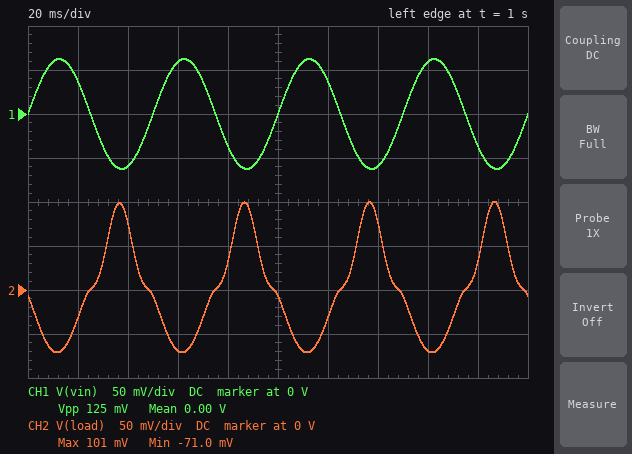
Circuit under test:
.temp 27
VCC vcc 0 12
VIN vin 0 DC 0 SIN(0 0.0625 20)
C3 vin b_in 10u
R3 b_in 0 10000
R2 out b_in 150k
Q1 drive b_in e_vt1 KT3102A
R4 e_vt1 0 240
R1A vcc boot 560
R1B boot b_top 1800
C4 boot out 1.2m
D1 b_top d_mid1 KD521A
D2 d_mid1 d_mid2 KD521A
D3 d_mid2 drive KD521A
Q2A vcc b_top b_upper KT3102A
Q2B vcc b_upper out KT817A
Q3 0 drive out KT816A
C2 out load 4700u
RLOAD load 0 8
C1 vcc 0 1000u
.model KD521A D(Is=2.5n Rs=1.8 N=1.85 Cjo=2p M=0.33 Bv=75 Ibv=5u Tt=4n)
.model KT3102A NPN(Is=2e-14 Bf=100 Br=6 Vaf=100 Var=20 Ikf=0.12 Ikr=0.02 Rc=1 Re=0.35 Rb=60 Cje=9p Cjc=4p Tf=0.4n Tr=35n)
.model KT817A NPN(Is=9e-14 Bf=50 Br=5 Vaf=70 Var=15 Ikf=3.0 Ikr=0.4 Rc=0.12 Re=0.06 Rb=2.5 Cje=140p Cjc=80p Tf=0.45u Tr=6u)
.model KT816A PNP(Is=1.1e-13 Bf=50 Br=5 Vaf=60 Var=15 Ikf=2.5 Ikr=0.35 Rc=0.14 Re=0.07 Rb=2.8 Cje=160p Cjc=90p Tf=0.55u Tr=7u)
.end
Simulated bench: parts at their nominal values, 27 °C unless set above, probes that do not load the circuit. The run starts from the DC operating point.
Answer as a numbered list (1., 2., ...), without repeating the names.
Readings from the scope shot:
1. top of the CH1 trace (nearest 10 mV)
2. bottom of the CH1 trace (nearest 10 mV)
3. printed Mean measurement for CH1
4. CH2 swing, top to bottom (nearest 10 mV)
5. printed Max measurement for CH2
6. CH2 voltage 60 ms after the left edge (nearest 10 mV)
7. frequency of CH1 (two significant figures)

1. 60 mV
2. -60 mV
3. 0.00 V
4. 170 mV
5. 101 mV
6. -70 mV
7. 20 Hz
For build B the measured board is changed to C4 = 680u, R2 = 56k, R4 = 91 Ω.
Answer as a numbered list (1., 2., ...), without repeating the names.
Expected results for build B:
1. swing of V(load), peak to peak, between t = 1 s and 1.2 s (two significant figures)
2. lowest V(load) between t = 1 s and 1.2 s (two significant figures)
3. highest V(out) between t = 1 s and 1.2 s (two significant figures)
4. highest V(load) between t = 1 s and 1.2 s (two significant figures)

1. 1.3 V
2. -380 mV
3. 7.8 V
4. 970 mV
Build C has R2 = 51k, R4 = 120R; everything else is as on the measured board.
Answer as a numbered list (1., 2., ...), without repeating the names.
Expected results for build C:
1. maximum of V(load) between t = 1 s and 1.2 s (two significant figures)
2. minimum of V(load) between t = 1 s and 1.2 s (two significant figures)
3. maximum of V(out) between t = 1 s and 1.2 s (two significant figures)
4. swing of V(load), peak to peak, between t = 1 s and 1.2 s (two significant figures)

1. 560 mV
2. -280 mV
3. 7.2 V
4. 840 mV
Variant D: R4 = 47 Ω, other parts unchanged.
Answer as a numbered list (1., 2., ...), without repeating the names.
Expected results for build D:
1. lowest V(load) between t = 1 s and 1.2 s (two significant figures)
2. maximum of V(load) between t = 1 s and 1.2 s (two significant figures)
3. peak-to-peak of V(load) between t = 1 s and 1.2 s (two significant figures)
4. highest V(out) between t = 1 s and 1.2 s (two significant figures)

1. -300 mV
2. 430 mV
3. 730 mV
4. 11 V
